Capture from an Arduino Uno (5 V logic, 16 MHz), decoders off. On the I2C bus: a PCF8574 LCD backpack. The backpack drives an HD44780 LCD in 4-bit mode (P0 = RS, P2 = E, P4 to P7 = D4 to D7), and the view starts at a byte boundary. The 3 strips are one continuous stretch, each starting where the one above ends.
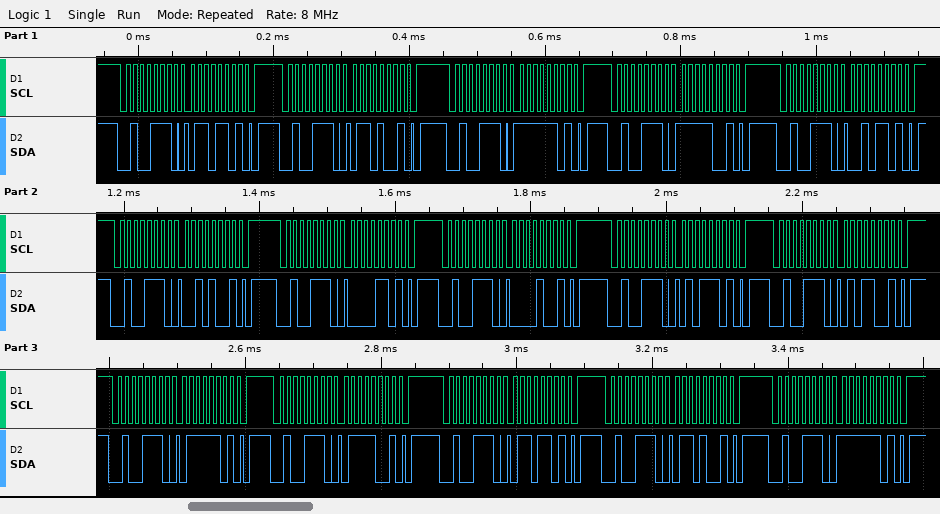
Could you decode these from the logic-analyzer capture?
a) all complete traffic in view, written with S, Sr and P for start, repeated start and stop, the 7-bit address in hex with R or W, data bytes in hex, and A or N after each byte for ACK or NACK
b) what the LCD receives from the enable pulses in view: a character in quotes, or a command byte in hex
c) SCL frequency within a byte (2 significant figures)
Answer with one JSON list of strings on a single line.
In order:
["S 27W A 6D A P S 27W A 69 A P S 27W A FD A P S 27W A F9 A P S 27W A 2D A P S 27W A 29 A P S 27W A 0D A P S 27W A 09 A P S 27W A 5D A P S 27W A 59 A P S 27W A 7D A P S 27W A 79 A P S 27W A 6D A P S 27W A 69 A P S 27W A FD A P", "'o' ' ' 'W'", "100 kHz"]
